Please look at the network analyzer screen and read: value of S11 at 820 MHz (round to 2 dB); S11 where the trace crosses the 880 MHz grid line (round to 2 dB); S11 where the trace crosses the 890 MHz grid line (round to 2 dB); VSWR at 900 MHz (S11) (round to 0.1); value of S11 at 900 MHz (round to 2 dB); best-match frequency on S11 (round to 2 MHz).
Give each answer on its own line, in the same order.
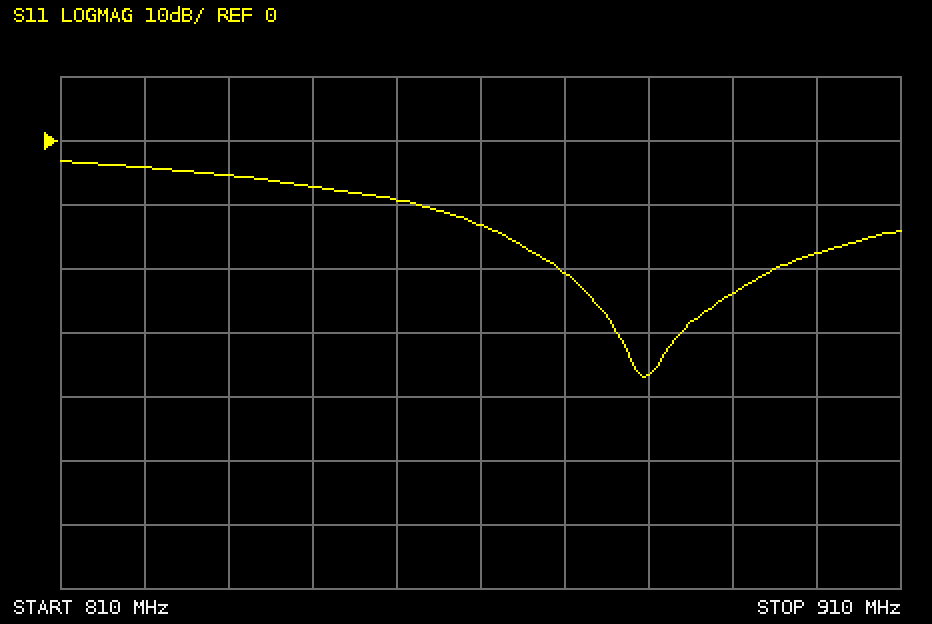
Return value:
-4 dB
-36 dB
-24 dB
1.3
-18 dB
880 MHz
